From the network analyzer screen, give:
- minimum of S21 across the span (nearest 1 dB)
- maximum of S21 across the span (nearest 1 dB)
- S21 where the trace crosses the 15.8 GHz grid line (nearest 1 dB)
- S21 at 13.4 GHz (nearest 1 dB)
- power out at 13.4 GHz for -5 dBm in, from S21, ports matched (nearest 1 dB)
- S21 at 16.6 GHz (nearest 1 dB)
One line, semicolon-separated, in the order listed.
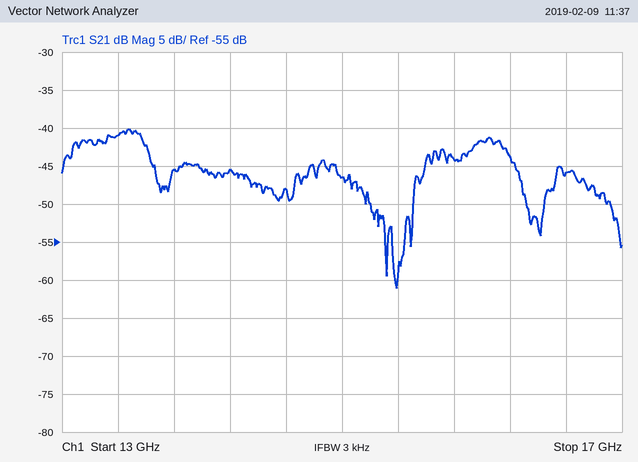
-61 dB; -40 dB; -44 dB; -41 dB; -46 dBm; -46 dB
